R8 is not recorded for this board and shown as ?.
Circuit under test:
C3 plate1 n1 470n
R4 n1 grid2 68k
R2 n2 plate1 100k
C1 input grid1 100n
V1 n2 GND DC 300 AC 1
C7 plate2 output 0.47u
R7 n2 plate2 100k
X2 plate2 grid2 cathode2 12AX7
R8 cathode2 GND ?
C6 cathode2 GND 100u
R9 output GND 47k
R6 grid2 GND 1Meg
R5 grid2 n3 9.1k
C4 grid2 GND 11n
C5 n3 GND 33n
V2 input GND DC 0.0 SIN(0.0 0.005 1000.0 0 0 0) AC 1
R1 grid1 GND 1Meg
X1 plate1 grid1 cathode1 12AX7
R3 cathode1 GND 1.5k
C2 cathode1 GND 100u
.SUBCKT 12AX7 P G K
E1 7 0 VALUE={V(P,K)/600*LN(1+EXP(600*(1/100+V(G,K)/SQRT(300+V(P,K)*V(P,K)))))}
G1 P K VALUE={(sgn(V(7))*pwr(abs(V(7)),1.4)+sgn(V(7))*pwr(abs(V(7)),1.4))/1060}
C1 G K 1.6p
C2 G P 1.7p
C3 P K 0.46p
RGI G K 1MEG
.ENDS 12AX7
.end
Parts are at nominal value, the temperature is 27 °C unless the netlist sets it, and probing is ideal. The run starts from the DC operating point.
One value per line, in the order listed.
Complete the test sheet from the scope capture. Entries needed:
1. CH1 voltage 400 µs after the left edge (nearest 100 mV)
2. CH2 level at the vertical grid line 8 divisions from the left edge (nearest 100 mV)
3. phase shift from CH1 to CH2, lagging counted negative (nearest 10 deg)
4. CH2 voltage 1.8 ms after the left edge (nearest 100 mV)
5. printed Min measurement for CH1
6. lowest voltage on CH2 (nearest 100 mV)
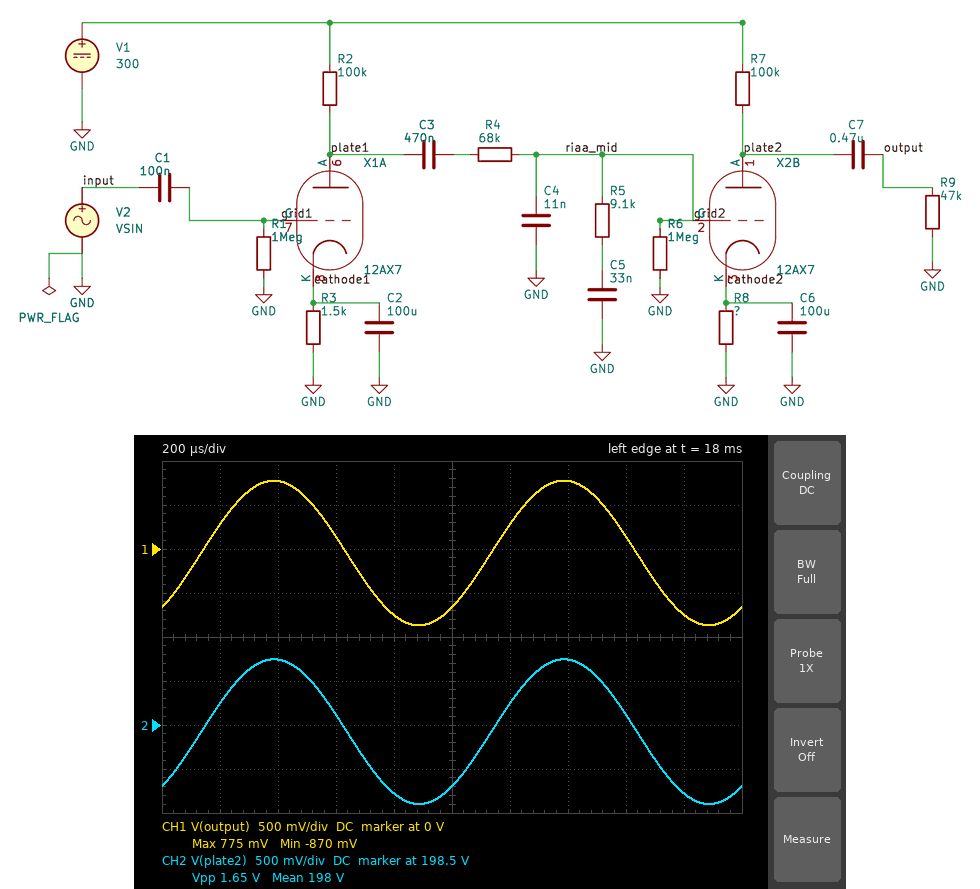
800 mV
198.6 V
0 deg
197.7 V
-870 mV
197.6 V
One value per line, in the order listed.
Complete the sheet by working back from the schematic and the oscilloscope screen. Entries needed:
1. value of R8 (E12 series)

2.7 kΩ
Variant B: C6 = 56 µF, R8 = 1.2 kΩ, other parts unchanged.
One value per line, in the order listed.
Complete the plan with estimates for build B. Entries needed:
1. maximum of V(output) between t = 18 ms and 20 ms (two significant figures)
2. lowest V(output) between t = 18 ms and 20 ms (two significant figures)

880 mV
-980 mV
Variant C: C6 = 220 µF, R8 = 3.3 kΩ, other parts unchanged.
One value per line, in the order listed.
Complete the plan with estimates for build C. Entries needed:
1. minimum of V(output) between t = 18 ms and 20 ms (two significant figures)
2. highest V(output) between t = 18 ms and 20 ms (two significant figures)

-830 mV
740 mV
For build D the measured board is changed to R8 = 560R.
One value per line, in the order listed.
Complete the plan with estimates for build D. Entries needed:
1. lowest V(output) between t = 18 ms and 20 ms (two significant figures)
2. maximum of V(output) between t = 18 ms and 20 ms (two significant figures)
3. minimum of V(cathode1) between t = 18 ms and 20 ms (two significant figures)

-1.0 V
930 mV
1.9 V
